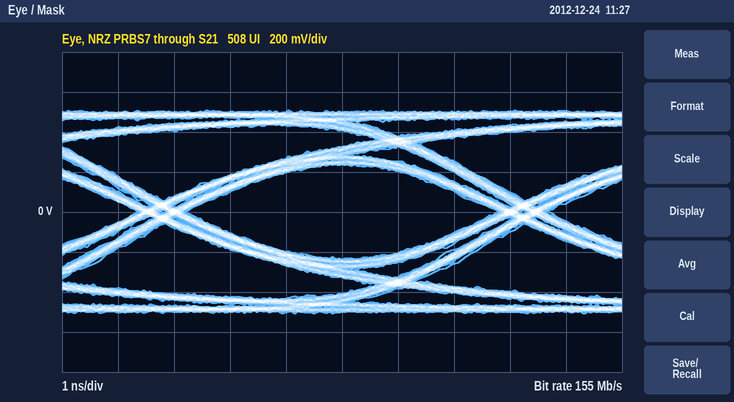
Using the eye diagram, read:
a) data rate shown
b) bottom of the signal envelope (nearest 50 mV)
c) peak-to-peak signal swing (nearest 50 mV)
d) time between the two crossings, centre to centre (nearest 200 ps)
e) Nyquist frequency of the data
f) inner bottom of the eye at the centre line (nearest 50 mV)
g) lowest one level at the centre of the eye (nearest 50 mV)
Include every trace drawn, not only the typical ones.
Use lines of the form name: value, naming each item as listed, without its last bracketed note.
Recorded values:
data rate shown: 155 Mb/s
bottom of the signal envelope: -500 mV
peak-to-peak signal swing: 1.00 V
time between the two crossings, centre to centre: 6.4 ns
Nyquist frequency of the data: 77.5 MHz
inner bottom of the eye at the centre line: -250 mV
lowest one level at the centre of the eye: 250 mV
